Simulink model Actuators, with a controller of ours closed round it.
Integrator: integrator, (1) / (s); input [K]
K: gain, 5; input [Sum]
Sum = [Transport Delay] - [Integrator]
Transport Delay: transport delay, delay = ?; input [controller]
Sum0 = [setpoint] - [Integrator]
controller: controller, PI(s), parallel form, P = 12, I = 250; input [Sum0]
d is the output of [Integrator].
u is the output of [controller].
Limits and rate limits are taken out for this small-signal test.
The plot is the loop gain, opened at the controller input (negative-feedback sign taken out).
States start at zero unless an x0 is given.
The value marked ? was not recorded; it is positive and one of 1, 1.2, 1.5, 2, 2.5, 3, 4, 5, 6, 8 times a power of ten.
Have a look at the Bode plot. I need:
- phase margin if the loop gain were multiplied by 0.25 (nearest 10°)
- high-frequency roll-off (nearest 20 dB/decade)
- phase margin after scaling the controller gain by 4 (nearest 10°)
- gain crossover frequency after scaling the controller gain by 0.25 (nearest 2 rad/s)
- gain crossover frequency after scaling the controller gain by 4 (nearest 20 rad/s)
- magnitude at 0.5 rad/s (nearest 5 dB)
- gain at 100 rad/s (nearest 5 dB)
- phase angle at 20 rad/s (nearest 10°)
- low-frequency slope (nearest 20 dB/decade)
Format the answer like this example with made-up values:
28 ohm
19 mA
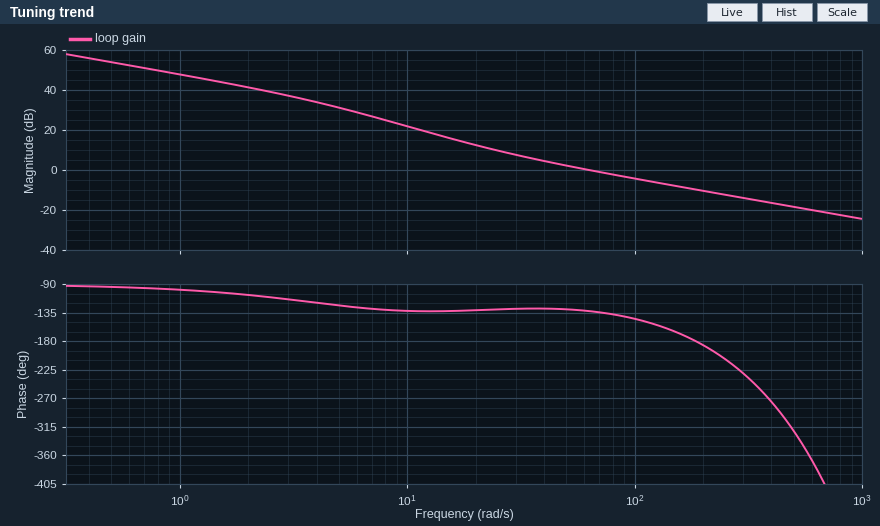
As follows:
50°
-20 dB/decade
-20°
20 rad/s
240 rad/s
55 dB
-5 dB
-130°
-20 dB/decade
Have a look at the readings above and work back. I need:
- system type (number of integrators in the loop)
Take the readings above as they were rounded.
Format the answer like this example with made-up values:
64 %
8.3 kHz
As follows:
1
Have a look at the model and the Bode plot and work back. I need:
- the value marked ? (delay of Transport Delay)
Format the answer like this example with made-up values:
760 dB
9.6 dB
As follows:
0.008
